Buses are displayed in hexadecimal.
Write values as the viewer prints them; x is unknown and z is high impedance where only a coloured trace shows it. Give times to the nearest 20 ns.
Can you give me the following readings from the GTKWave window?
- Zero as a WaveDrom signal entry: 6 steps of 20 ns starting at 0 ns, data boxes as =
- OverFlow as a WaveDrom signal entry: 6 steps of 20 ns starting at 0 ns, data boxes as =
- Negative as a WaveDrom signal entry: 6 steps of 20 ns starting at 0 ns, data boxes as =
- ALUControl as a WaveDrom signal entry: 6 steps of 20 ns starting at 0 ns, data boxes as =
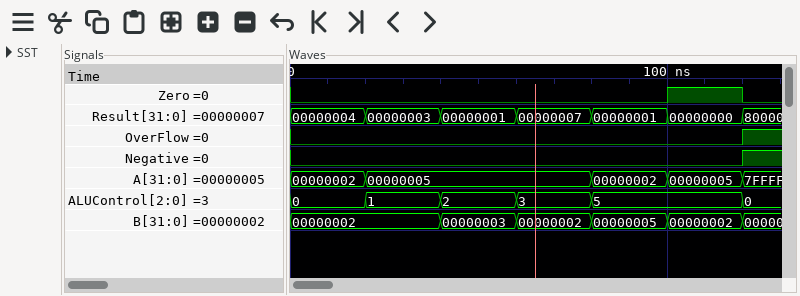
{name: 'Zero', wave: '0....1'}
{name: 'OverFlow', wave: '0.....'}
{name: 'Negative', wave: '0.....'}
{name: 'ALUControl', wave: '=====.', data: '0 1 2 3 5'}
